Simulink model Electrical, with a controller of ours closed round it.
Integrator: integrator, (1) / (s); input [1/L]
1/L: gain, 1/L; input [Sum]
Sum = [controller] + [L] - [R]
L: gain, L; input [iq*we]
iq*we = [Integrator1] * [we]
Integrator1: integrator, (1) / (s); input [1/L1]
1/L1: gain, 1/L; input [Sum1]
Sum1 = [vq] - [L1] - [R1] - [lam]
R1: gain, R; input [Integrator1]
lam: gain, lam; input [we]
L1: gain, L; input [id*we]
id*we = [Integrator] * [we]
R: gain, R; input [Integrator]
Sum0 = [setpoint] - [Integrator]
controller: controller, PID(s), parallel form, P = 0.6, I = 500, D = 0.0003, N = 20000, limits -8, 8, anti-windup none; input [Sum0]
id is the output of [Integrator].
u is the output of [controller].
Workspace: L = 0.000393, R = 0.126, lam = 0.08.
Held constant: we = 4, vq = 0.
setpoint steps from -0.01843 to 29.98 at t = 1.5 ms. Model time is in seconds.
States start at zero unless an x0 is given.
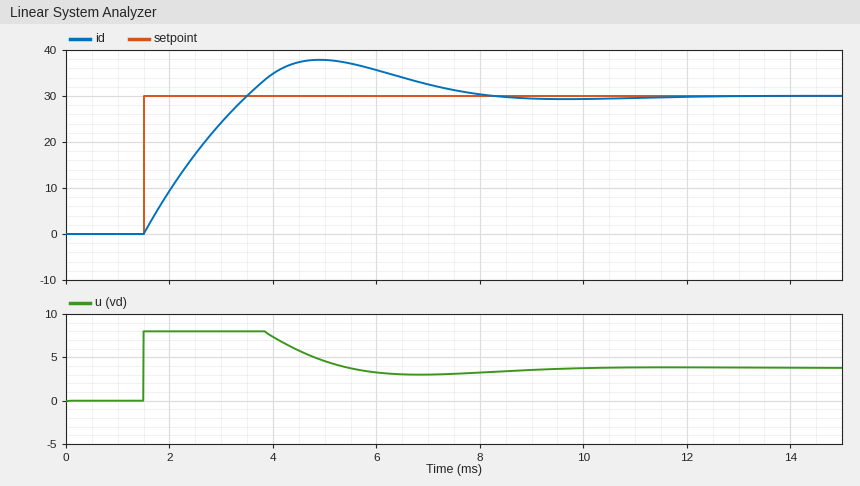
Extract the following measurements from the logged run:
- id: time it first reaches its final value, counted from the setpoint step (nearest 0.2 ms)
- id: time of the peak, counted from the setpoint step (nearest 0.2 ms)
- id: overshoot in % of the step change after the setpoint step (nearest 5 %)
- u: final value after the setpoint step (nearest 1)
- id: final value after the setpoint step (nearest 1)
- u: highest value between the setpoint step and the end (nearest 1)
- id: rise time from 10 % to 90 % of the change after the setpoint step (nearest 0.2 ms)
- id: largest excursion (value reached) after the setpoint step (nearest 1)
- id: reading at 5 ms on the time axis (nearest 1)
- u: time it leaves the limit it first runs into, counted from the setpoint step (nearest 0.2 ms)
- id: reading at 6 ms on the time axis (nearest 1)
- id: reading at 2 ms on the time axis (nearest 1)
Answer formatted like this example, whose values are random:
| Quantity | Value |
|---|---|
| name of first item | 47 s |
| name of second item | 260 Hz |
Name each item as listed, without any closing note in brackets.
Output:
| Quantity | Value |
|---|---|
| id: time it first reaches its final value, counted from the setpoint step | 2.0 ms |
| id: time of the peak, counted from the setpoint step | 3.4 ms |
| id: overshoot in % of the step change after the setpoint step | 25 % |
| u: final value after the setpoint step | 4 |
| id: final value after the setpoint step | 30 |
| u: highest value between the setpoint step and the end | 8 |
| id: rise time from 10 % to 90 % of the change after the setpoint step | 1.6 ms |
| id: largest excursion (value reached) after the setpoint step | 38 |
| id: reading at 5 ms on the time axis | 38 |
| u: time it leaves the limit it first runs into, counted from the setpoint step | 2.4 ms |
| id: reading at 6 ms on the time axis | 36 |
| id: reading at 2 ms on the time axis | 9 |
